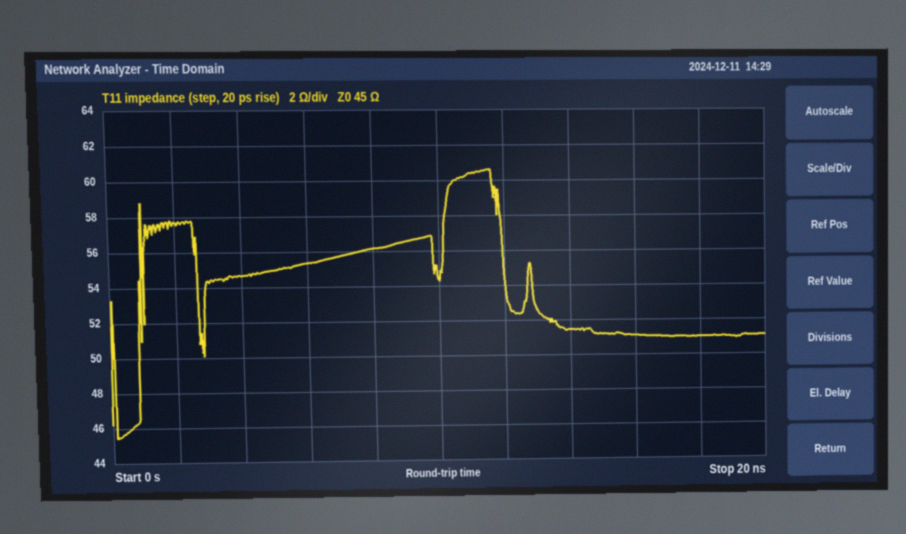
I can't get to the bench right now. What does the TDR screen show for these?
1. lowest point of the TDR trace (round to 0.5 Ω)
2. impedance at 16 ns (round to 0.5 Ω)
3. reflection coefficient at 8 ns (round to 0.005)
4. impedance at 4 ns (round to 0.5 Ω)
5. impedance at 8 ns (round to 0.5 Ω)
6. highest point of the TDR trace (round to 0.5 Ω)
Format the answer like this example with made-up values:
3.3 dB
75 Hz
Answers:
45.5 Ω
51.0 Ω
+0.110
54.5 Ω
56.0 Ω
60.5 Ω
